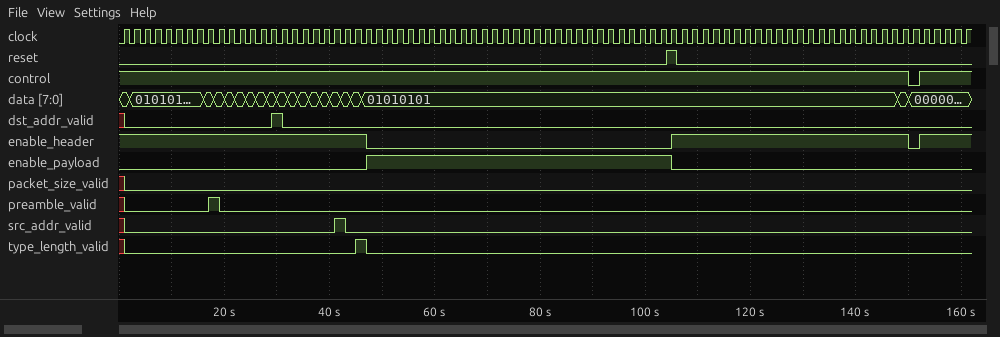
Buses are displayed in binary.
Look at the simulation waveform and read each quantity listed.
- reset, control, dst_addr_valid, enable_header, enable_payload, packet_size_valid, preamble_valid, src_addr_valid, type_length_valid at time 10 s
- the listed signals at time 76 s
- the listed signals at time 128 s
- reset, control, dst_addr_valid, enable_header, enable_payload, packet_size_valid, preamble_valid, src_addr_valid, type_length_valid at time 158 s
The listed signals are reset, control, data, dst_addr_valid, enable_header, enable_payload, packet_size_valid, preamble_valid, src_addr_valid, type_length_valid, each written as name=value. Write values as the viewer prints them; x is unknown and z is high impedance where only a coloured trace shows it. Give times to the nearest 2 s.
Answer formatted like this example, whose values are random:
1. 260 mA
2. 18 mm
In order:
1. reset=0, control=1, dst_addr_valid=0, enable_header=1, enable_payload=0, packet_size_valid=0, preamble_valid=0, src_addr_valid=0, type_length_valid=0
2. reset=0, control=1, data=01010101, dst_addr_valid=0, enable_header=0, enable_payload=1, packet_size_valid=0, preamble_valid=0, src_addr_valid=0, type_length_valid=0
3. reset=0, control=1, data=01010101, dst_addr_valid=0, enable_header=1, enable_payload=0, packet_size_valid=0, preamble_valid=0, src_addr_valid=0, type_length_valid=0
4. reset=0, control=1, dst_addr_valid=0, enable_header=1, enable_payload=0, packet_size_valid=0, preamble_valid=0, src_addr_valid=0, type_length_valid=0
